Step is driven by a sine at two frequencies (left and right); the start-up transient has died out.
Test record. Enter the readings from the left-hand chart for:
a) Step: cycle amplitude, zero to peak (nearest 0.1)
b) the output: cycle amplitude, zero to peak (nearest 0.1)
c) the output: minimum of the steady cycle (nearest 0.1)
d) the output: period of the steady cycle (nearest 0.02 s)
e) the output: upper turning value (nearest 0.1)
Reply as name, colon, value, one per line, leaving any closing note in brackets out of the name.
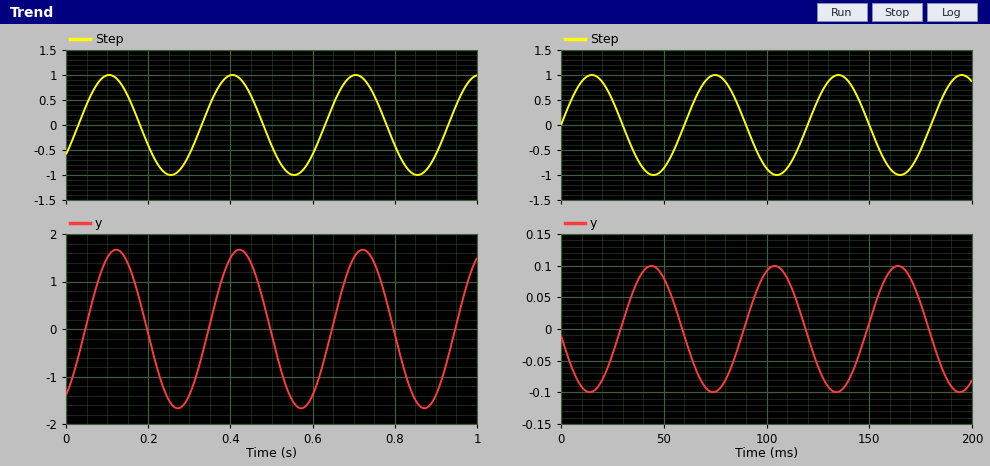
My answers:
Step: cycle amplitude, zero to peak: 1.0
the output: cycle amplitude, zero to peak: 1.7
the output: minimum of the steady cycle: -1.7
the output: period of the steady cycle: 0.30 s
the output: upper turning value: 1.7
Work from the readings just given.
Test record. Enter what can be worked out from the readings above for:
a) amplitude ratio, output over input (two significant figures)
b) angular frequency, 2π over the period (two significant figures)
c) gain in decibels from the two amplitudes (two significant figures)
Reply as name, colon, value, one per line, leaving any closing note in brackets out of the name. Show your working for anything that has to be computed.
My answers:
amplitude ratio, output over input: 1.7 / 1 = 1.7
angular frequency, 2π over the period: 2π / 0.3 = 21 rad/s
gain in decibels from the two amplitudes: 20 log10(1.7 / 1) = 4.6 dB
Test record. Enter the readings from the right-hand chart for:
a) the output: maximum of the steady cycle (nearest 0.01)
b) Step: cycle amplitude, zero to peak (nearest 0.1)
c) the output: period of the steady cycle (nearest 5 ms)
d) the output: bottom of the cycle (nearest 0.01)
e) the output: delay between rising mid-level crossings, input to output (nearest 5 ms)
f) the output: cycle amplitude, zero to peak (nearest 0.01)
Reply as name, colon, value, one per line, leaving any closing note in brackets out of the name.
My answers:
the output: maximum of the steady cycle: 0.10
Step: cycle amplitude, zero to peak: 1.0
the output: period of the steady cycle: 60 ms
the output: bottom of the cycle: -0.10
the output: delay between rising mid-level crossings, input to output: 30 ms
the output: cycle amplitude, zero to peak: 0.10
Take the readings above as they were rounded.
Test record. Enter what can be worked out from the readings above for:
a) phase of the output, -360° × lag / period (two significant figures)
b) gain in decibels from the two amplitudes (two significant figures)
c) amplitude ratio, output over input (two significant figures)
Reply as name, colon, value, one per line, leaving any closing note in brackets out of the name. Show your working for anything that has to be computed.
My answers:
phase of the output, -360° × lag / period: -360 × 30 / 60 = -180°
gain in decibels from the two amplitudes: 20 log10(0.1 / 1) = -20 dB
amplitude ratio, output over input: 0.1 / 1 = 0.10
